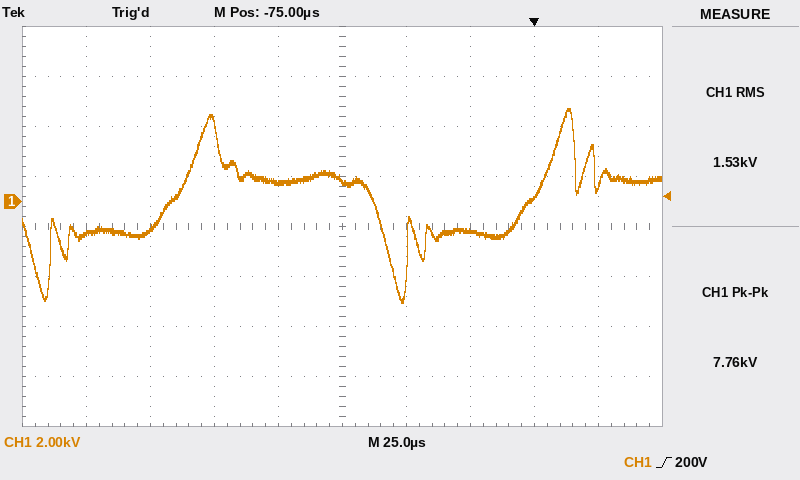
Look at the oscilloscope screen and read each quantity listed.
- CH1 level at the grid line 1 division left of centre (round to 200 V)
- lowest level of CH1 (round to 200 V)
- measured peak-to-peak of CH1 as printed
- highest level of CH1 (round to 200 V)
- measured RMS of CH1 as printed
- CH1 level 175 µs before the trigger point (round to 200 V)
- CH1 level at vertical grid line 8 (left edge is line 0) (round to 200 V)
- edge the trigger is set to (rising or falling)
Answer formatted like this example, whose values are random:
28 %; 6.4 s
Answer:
800 V; -4.0 kV; 7.76 kV; 3.8 kV; 1.53 kV; -1.2 kV; 200 V; rising
